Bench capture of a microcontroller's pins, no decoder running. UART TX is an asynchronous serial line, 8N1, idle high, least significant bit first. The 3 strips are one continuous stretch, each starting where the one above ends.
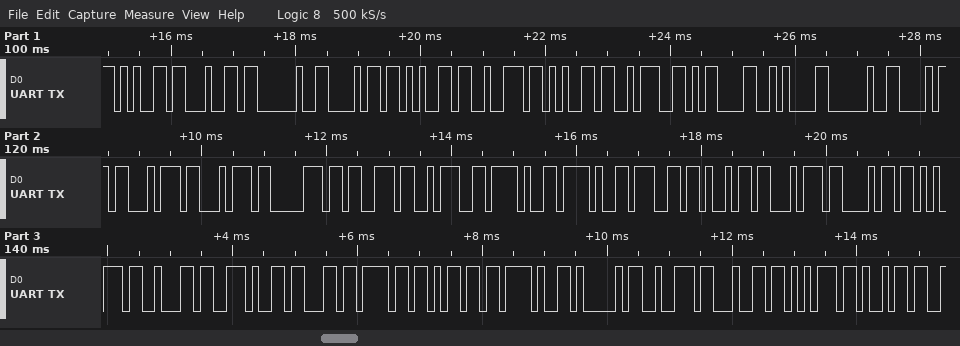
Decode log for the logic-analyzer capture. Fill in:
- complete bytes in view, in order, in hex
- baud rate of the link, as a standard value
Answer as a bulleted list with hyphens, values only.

- 0x65 0x64 0x20 0x68 0x65 0x72 0x65 0x3A 0x0D 0x0A 0x20 0x68 0x74 0x74 0x70 0x73 0x3A 0x2F 0x2F 0x67 0x69 0x74 0x68 0x75 0x62 0x2E 0x63 0x6F 0x6D 0x2F 0x41 0x72 0x64 0x75 0x69
- 9600 baud
